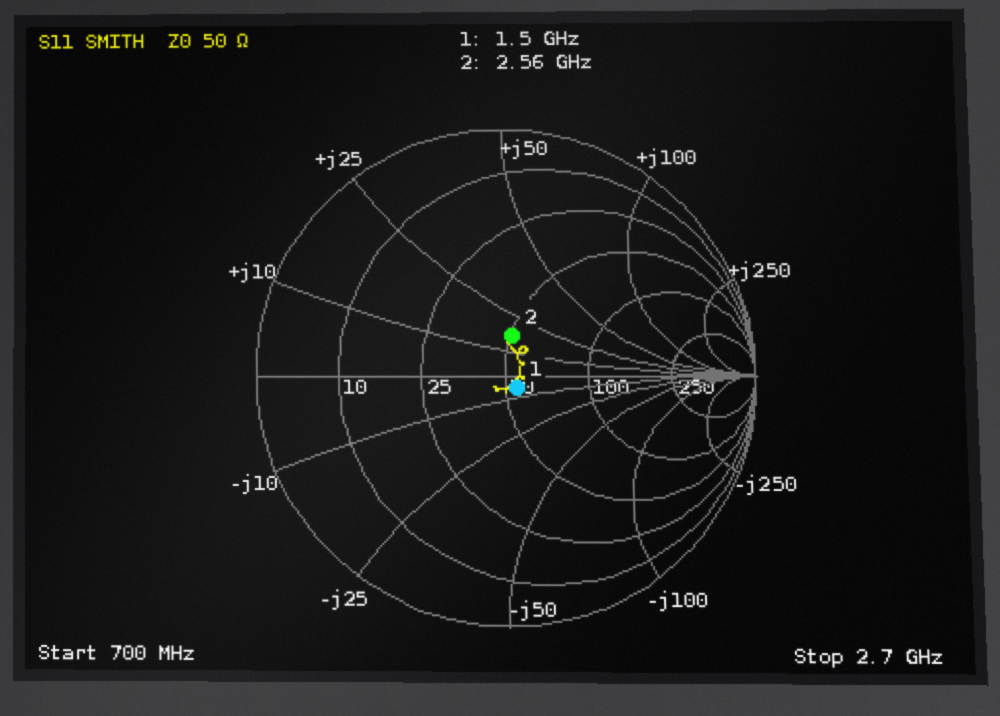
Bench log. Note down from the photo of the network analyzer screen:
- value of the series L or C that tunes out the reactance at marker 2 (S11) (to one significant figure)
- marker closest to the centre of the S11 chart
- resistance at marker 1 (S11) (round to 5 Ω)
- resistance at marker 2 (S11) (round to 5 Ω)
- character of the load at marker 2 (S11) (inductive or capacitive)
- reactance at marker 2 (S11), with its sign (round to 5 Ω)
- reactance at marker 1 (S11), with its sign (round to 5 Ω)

4 pF
marker 1
55 Ω
50 Ω
inductive
+15 Ω
-5 Ω
